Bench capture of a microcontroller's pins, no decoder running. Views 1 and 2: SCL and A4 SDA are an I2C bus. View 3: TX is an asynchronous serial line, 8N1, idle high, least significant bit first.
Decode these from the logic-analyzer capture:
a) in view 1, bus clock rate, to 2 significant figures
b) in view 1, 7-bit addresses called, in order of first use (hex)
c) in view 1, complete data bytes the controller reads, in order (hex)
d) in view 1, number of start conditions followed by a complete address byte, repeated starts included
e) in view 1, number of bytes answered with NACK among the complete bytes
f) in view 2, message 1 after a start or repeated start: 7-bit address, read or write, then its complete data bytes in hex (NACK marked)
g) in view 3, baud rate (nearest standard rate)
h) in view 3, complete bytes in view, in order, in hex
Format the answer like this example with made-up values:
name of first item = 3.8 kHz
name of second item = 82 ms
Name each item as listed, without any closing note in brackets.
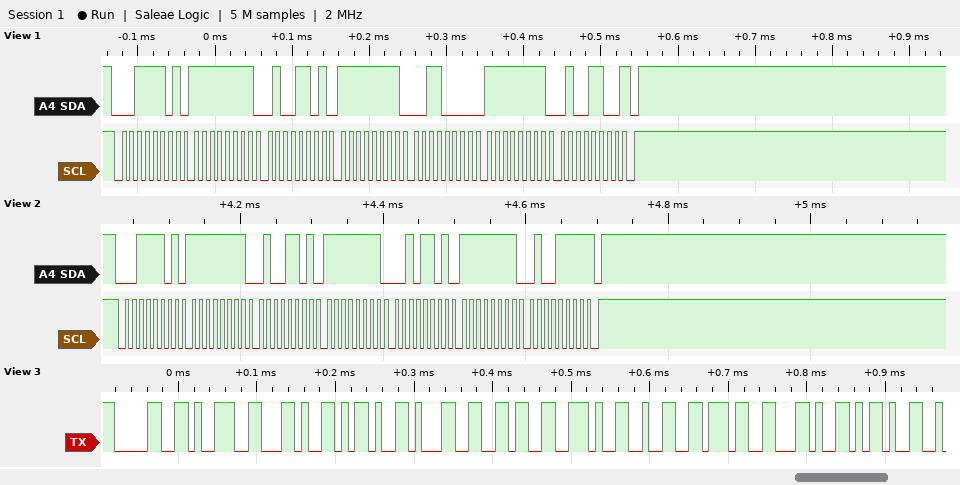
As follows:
in view 1, bus clock rate, to 2 significant figures = 100 kHz
in view 1, 7-bit addresses called, in order of first use = 0x1E
in view 1, complete data bytes the controller reads, in order = FF 4D FF 30 FF 4C
in view 1, number of start conditions followed by a complete address byte, repeated starts included = 1
in view 1, number of bytes answered with NACK among the complete bytes = 1
in view 2, message 1 after a start or repeated start: 7-bit address, read or write, then its complete data bytes in hex = 0x1E read: FF 4D FF 2D FF 4F NACK
in view 3, baud rate = 115200 baud
in view 3, complete bytes in view, in order, in hex = 30 39 2C 2D 31 36 2E 32 37 2C 2D
